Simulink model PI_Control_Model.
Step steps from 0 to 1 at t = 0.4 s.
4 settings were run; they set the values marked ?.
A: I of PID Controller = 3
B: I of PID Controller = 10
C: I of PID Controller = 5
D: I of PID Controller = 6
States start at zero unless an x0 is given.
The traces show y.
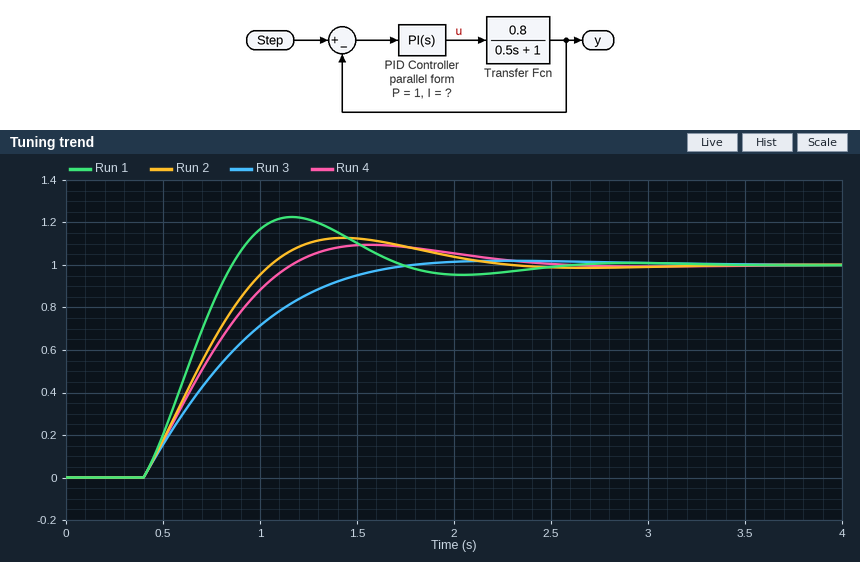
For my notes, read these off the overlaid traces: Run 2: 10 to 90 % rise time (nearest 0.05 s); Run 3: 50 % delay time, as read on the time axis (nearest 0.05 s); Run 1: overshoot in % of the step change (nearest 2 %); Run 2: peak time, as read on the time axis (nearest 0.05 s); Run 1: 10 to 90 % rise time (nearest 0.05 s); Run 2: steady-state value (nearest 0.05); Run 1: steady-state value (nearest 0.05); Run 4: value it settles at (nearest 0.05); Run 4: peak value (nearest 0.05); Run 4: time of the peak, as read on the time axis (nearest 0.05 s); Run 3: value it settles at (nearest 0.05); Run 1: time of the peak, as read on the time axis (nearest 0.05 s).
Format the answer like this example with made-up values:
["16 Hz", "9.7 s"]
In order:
["0.50 s", "0.75 s", "22 %", "1.45 s", "0.35 s", "1.00", "1.00", "1.00", "1.10", "1.55 s", "1.00", "1.15 s"]
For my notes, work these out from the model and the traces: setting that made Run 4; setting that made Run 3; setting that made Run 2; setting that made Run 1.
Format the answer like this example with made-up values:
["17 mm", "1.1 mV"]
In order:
["C", "A", "D", "B"]
